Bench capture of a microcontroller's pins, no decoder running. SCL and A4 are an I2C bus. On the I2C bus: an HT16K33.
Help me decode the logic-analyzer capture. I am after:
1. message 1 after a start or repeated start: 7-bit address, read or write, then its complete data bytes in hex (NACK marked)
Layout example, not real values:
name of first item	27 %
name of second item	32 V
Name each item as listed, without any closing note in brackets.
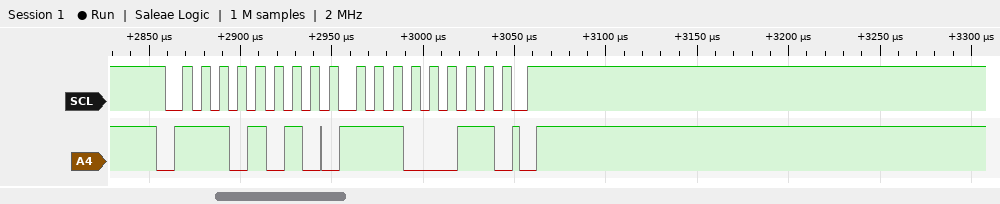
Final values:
message 1 after a start or repeated start: 7-bit address, read or write, then its complete data bytes in hex	0x75 write: E3
